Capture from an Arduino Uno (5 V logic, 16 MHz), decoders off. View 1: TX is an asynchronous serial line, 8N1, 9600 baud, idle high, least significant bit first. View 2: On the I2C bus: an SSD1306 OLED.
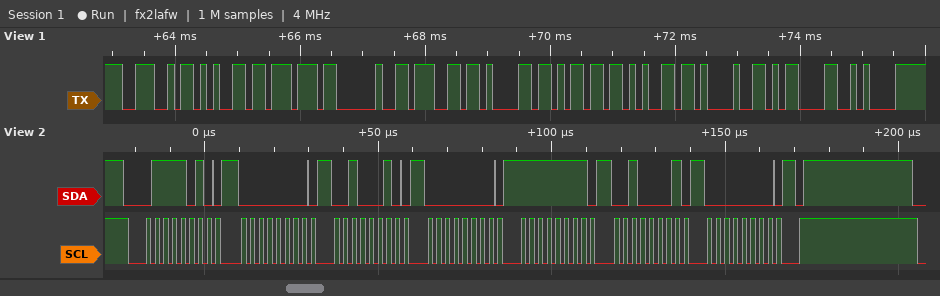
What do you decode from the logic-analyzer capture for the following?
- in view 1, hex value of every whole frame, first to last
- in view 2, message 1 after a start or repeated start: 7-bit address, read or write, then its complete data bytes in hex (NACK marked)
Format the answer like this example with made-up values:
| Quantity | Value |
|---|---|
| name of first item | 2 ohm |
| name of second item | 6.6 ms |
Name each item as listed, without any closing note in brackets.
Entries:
| Quantity | Value |
|---|---|
| in view 1, hex value of every whole frame, first to last | 4E 65 77 20 67 61 6D 65 21 0D 0A |
| in view 2, message 1 after a start or repeated start: 7-bit address, read or write, then its complete data bytes in hex | 0x3D write: 00 22 00 FF 21 00 |
